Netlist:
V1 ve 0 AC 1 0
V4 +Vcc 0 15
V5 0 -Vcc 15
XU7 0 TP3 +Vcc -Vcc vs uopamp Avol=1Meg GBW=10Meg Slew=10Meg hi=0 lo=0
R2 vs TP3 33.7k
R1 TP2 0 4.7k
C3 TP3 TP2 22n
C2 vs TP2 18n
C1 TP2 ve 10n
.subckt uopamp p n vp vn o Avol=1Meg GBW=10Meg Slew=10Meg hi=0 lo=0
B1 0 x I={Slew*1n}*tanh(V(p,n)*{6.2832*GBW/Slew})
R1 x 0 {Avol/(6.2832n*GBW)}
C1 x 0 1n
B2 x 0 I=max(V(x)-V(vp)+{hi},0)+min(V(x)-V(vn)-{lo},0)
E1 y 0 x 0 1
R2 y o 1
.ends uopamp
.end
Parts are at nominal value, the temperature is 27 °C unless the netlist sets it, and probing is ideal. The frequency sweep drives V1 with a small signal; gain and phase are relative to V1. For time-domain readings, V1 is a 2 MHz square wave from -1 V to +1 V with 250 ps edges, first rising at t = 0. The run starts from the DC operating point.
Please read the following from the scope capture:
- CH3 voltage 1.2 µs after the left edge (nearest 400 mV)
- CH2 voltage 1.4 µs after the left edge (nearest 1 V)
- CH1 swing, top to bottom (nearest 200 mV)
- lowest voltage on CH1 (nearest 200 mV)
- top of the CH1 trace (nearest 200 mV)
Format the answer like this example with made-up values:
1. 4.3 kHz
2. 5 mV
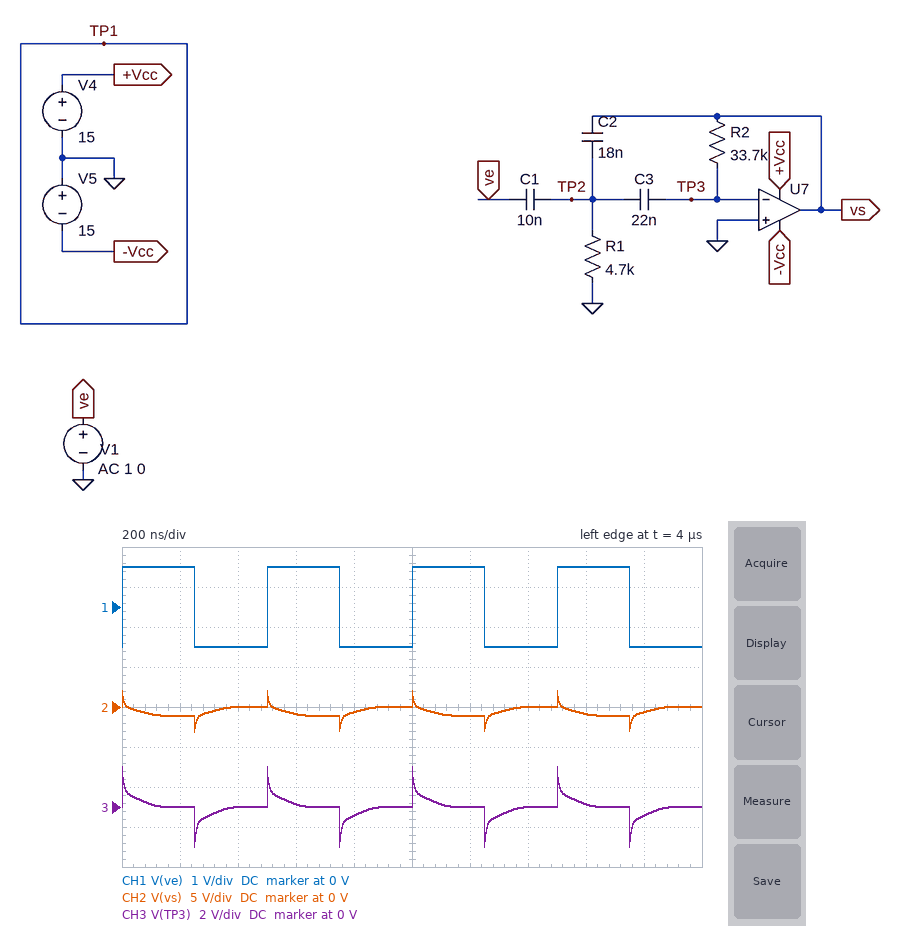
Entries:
1. 0 V
2. 0 V
3. 2.0 V
4. -1.0 V
5. 1.0 V
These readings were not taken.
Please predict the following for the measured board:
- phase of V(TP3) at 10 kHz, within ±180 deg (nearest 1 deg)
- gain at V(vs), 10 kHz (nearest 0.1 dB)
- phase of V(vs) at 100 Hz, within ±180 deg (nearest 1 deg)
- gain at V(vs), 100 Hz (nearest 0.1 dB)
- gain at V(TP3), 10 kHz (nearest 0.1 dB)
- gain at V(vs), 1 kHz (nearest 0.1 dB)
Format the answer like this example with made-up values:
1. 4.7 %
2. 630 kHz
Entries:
1. 93 deg
2. -5.1 dB
3. -9 deg
4. -37.1 dB
5. -65.1 dB
6. -3.6 dB
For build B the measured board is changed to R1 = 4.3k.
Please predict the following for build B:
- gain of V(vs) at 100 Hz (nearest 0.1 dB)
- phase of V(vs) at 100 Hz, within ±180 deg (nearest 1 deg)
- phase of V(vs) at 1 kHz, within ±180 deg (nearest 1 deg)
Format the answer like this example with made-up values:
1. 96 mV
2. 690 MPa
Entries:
1. -37.9 dB
2. -8 deg
3. -133 deg
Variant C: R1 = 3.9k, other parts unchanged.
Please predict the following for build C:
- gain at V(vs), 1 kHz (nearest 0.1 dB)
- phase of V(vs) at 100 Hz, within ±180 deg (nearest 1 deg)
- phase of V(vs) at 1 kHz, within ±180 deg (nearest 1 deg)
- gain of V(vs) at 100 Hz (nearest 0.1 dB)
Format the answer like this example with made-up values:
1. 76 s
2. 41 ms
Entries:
1. -3.0 dB
2. -7 deg
3. -131 deg
4. -38.7 dB
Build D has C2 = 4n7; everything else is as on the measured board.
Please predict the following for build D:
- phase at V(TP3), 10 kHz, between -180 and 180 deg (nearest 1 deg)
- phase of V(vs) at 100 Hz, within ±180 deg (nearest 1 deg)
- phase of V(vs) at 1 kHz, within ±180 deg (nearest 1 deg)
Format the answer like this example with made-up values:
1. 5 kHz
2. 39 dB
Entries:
1. 99 deg
2. -6 deg
3. -72 deg
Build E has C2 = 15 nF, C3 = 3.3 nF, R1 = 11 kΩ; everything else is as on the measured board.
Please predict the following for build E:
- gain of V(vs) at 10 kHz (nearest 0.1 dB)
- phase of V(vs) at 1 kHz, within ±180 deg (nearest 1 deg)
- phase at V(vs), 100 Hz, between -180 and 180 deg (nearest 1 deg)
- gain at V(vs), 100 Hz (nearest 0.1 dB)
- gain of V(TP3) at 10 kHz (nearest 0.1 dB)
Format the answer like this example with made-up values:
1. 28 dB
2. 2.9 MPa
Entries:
1. -3.7 dB
2. -82 deg
3. -11 deg
4. -46.4 dB
5. -63.7 dB
